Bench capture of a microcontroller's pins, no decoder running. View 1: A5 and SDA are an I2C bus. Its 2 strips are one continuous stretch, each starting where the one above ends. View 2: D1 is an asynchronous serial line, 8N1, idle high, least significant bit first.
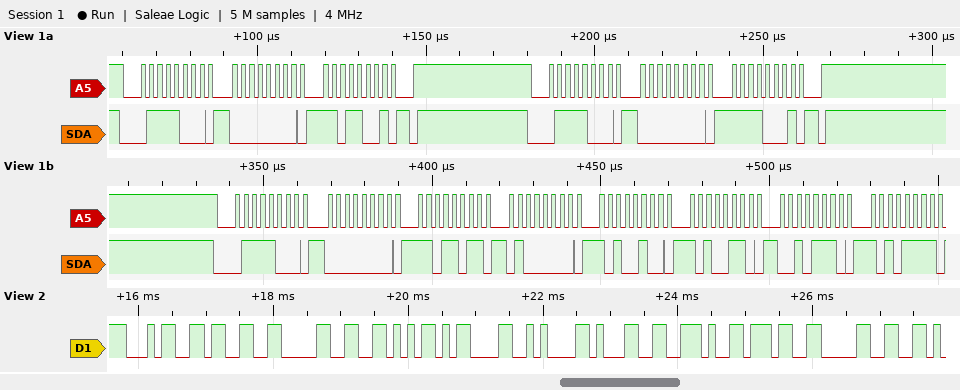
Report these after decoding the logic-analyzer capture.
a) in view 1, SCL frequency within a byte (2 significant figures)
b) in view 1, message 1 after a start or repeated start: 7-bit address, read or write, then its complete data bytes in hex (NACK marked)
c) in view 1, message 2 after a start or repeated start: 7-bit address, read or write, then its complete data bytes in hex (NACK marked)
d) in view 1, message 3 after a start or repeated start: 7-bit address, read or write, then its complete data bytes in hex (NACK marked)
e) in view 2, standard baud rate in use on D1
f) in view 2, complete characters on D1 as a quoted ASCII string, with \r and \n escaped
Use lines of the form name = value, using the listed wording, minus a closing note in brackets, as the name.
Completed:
in view 1, SCL frequency within a byte = 400 kHz
in view 1, message 1 after a start or repeated start: 7-bit address, read or write, then its complete data bytes in hex = 0x3C write: 00 D9
in view 1, message 2 after a start or repeated start: 7-bit address, read or write, then its complete data bytes in hex = 0x3C write: 00 F1
in view 1, message 3 after a start or repeated start: 7-bit address, read or write, then its complete data bytes in hex = 0x3C write: 00 DB 40 A4 A6 2E AF
in view 2, standard baud rate in use on D1 = 9600 baud
in view 2, complete characters on D1 as a quoted ASCII string, with \r and \n escaped = "430V\r\n1.70"
